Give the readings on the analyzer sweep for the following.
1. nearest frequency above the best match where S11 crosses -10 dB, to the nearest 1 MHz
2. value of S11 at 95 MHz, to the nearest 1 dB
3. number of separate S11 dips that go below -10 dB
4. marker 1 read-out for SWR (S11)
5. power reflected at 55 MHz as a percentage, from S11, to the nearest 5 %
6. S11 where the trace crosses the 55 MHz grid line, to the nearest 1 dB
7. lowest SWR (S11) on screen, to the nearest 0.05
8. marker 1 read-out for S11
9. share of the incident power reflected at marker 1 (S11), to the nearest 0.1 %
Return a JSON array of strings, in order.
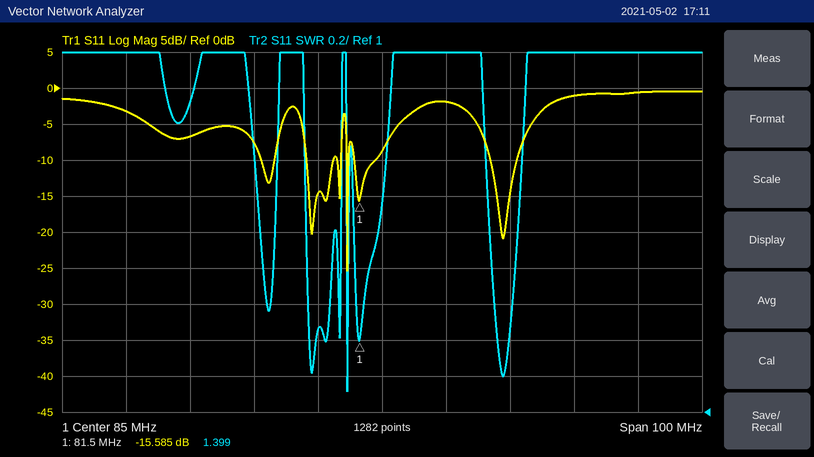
["80 MHz", "-2 dB", "6", "1.399", "20 %", "-7 dB", "1.10", "-15.585 dB", "2.8 %"]
